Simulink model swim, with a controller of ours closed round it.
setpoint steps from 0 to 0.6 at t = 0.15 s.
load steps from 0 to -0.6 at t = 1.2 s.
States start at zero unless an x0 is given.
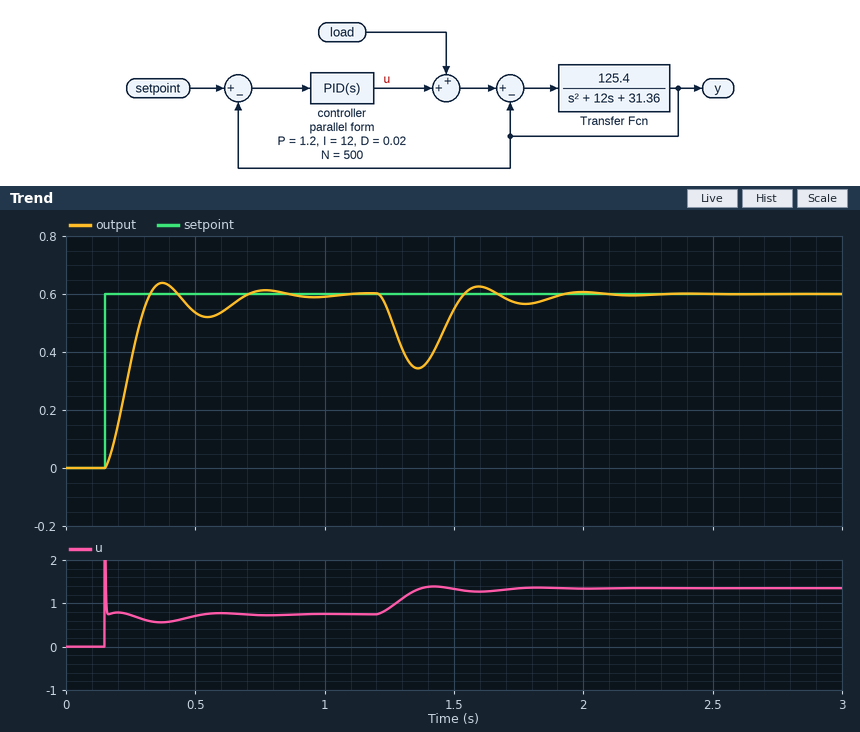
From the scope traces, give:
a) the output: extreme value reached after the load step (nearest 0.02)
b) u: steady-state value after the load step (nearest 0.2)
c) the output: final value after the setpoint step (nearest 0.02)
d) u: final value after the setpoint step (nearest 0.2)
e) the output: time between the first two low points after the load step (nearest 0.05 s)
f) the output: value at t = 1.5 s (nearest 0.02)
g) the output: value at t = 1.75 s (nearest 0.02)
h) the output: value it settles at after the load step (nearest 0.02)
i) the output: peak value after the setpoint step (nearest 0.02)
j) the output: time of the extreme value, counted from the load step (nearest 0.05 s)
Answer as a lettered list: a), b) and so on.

a) 0.34
b) 1.4
c) 0.60
d) 0.8
e) 0.40 s
f) 0.54
g) 0.56
h) 0.60
i) 0.64
j) 0.15 s
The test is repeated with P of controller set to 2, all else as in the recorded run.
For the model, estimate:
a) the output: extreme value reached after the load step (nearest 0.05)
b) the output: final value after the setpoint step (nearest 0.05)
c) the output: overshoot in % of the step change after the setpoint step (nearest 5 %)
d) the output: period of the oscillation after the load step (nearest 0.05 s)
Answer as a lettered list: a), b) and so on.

a) 0.40
b) 0.60
c) 10 %
d) 0.35 s
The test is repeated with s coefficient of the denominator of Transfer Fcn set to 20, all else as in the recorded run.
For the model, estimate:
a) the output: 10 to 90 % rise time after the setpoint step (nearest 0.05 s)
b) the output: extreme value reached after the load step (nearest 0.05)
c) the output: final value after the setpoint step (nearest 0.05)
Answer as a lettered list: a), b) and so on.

a) 0.15 s
b) 0.40
c) 0.60
